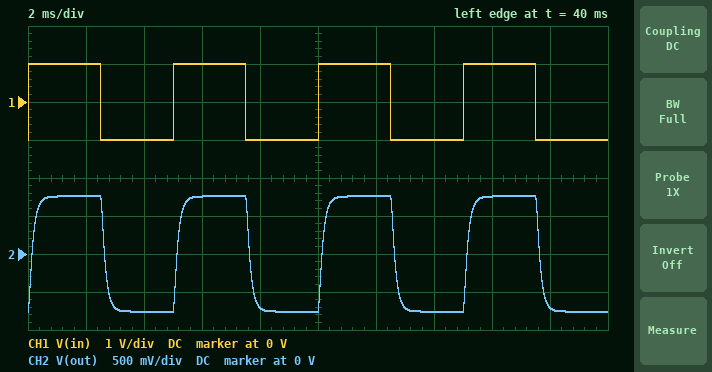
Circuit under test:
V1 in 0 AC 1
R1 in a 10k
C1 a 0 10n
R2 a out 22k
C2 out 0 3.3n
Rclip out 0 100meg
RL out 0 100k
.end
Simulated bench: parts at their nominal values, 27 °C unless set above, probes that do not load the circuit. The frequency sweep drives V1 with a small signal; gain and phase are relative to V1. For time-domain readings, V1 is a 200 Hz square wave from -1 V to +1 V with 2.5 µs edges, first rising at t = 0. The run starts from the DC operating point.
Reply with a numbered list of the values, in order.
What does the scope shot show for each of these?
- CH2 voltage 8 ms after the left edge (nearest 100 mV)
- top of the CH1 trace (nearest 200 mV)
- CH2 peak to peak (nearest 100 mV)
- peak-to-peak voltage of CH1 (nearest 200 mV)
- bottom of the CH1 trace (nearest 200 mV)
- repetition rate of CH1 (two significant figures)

1. -700 mV
2. 1.0 V
3. 1.5 V
4. 2.0 V
5. -1.0 V
6. 200 Hz
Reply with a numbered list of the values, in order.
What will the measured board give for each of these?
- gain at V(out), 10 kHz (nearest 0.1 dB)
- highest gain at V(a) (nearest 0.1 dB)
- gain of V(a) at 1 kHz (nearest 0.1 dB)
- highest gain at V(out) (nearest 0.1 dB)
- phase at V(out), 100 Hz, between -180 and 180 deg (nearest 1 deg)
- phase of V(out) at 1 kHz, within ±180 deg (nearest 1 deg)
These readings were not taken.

1. -29.8 dB
2. -0.7 dB
3. -2.6 dB
4. -2.4 dB
5. -6 deg
6. -54 deg
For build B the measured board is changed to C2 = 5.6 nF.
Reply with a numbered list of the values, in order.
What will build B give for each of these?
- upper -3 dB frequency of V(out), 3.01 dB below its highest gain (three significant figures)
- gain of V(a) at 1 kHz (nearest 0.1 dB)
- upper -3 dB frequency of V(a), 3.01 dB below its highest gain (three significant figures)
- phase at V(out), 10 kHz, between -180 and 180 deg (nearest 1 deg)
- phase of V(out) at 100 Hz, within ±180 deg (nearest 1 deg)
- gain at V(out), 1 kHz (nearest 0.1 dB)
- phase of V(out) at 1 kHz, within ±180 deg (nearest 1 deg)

1. 841 Hz
2. -3.1 dB
3. 1.19 kHz
4. -158 deg
5. -8 deg
6. -6.3 dB
7. -66 deg
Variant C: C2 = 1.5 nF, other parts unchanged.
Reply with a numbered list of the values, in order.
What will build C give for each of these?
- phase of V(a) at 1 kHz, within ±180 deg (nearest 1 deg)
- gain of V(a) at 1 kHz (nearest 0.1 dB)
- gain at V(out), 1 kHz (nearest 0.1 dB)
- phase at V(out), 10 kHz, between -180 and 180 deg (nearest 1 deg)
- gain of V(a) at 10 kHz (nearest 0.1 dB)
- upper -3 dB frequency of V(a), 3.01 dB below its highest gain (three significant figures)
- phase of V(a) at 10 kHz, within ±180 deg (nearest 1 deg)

1. -32 deg
2. -2.2 dB
3. -4.1 dB
4. -138 deg
5. -16.4 dB
6. 1.54 kHz
7. -78 deg
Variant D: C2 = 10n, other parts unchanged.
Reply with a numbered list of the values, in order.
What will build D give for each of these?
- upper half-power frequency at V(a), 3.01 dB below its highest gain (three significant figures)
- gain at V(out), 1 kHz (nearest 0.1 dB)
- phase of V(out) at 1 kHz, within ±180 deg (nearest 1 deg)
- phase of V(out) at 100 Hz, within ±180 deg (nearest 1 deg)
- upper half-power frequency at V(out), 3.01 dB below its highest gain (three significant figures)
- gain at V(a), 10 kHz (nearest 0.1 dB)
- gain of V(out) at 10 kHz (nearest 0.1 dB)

1. 1.01 kHz
2. -9.0 dB
3. -81 deg
4. -12 deg
5. 555 Hz
6. -16.2 dB
7. -39.1 dB
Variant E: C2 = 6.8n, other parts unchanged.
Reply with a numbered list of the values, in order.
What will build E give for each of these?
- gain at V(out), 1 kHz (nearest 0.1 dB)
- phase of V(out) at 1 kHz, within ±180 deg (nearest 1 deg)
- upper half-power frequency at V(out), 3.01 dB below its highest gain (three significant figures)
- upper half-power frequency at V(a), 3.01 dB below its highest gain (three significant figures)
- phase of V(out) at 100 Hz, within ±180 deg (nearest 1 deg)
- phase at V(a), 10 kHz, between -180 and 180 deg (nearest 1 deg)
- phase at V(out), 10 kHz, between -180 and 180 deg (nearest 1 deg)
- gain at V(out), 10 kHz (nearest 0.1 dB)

1. -7.1 dB
2. -71 deg
3. 740 Hz
4. 1.13 kHz
5. -9 deg
6. -77 deg
7. -160 deg
8. -35.8 dB
